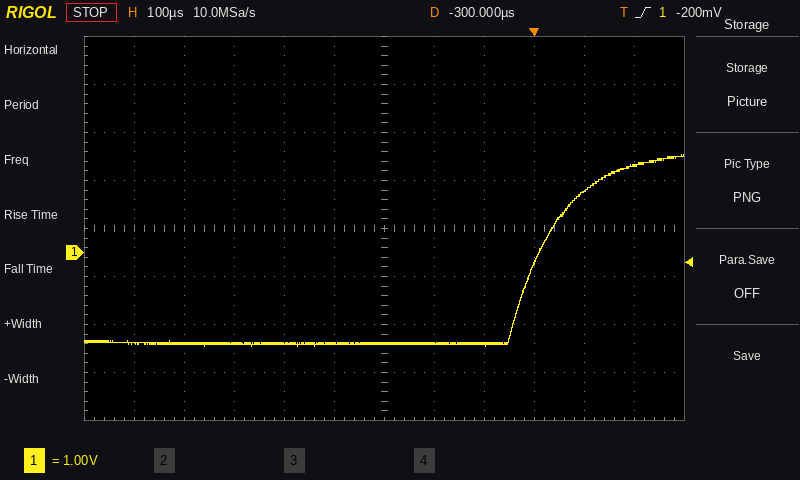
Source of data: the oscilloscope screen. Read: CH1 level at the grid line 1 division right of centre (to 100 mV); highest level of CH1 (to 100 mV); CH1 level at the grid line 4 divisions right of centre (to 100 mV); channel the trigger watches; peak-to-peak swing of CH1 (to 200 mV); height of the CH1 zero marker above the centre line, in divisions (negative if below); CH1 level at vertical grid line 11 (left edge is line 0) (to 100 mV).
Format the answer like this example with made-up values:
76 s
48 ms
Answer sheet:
-1.9 V
2.0 V
1.3 V
CH1
4.0 V
-0.5 div
1.8 V
